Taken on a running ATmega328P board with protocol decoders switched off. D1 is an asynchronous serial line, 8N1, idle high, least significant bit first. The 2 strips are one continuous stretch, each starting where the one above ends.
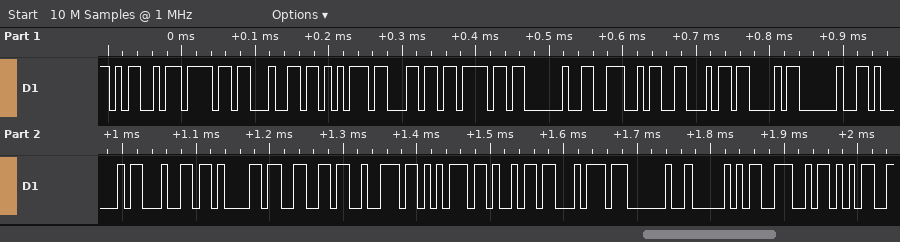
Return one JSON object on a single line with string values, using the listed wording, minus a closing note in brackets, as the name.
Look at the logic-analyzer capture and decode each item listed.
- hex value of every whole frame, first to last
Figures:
{"hex value of every whole frame, first to last": "0x4D 0x6F 0x64 0x75 0x6C 0x6F 0x20 0x4E 0x46 0x43 0x20 0x41 0x64 0x61 0x66 0x72 0x75 0x69 0x74 0x20 0x50 0x4E 0x35"}
